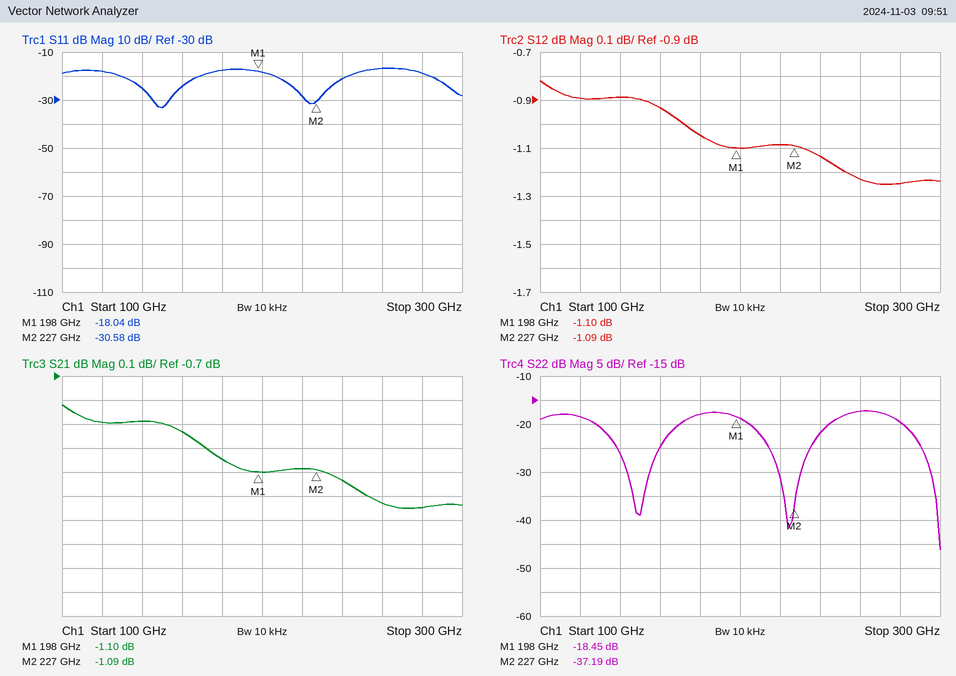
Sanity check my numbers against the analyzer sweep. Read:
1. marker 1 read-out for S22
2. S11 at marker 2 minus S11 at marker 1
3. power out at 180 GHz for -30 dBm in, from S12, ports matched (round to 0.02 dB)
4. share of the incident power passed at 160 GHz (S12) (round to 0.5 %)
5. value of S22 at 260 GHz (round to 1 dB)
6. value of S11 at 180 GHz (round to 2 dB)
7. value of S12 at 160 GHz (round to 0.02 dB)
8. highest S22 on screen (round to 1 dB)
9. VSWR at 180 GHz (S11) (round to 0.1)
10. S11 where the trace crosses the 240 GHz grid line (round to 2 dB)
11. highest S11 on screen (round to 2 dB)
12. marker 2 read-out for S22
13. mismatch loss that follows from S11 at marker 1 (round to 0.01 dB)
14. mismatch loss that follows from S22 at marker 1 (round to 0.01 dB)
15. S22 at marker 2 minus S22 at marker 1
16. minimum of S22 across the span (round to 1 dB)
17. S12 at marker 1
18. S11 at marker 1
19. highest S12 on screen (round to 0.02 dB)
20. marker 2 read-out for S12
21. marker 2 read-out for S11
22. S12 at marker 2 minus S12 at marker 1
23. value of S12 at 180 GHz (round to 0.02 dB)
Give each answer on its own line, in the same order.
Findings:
-18.45 dB
-12.54 dB
-31.04 dBm
80.5 %
-17 dB
-18 dB
-0.94 dB
-17 dB
1.3
-22 dB
-16 dB
-37.19 dB
0.07 dB
0.06 dB
-18.74 dB
-46 dB
-1.10 dB
-18.04 dB
-0.82 dB
-1.09 dB
-30.58 dB
0.01 dB
-1.04 dB
